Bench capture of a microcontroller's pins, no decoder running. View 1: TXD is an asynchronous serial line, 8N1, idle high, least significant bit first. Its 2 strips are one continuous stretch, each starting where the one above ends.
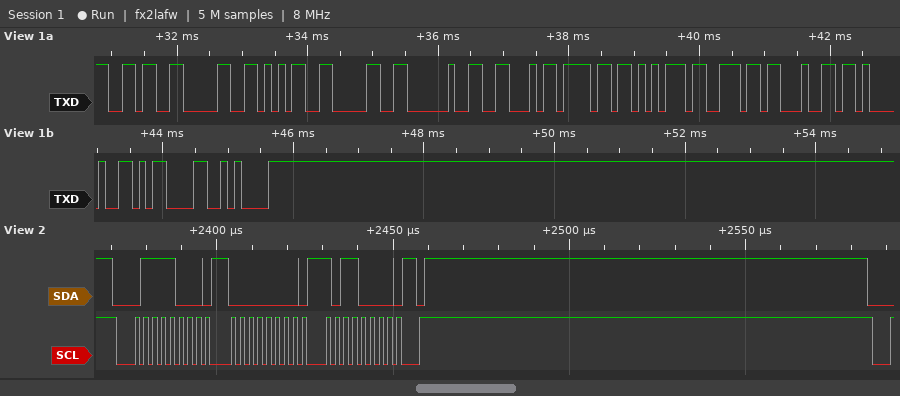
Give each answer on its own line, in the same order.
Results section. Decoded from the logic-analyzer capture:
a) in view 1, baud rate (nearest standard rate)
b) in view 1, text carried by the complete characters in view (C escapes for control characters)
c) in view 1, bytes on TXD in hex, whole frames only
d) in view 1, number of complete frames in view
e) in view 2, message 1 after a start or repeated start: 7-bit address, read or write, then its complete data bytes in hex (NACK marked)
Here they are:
9600 baud
"6050 Found!\r\n"
0x36 0x30 0x35 0x30 0x20 0x46 0x6F 0x75 0x6E 0x64 0x21 0x0D 0x0A
13
0x3C write: 00 B0
